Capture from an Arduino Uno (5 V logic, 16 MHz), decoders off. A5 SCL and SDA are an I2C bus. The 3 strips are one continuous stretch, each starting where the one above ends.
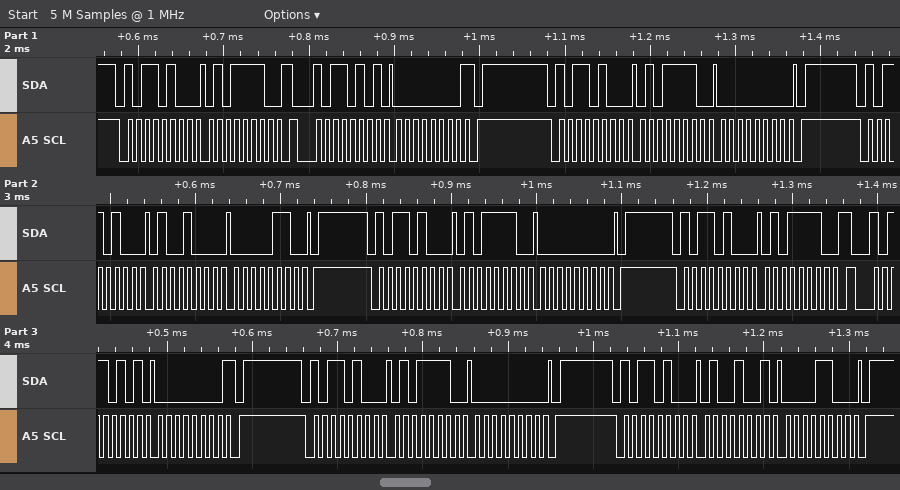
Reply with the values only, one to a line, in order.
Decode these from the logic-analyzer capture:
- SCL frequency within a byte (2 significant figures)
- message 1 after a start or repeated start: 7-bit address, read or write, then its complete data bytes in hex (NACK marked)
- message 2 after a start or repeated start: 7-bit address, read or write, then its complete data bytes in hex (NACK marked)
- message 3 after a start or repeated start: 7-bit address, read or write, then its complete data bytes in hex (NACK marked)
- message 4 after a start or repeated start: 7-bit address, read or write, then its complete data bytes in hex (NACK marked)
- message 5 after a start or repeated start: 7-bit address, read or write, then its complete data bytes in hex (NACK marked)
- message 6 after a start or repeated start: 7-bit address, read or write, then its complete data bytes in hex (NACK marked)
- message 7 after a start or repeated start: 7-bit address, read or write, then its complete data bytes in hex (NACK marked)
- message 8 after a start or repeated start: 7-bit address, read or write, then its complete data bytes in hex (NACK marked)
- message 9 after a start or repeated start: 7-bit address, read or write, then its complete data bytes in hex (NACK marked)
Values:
100 kHz
0x5A write: 5E
0x5A read: 00 NACK
0x5A write: 5E 00
0x5A write: 48 06
0x5A write: 5E 00
0x5A write: 5E
0x5A read: 00 NACK
0x5A write: 5E 00
0x5A write: 49 0C
